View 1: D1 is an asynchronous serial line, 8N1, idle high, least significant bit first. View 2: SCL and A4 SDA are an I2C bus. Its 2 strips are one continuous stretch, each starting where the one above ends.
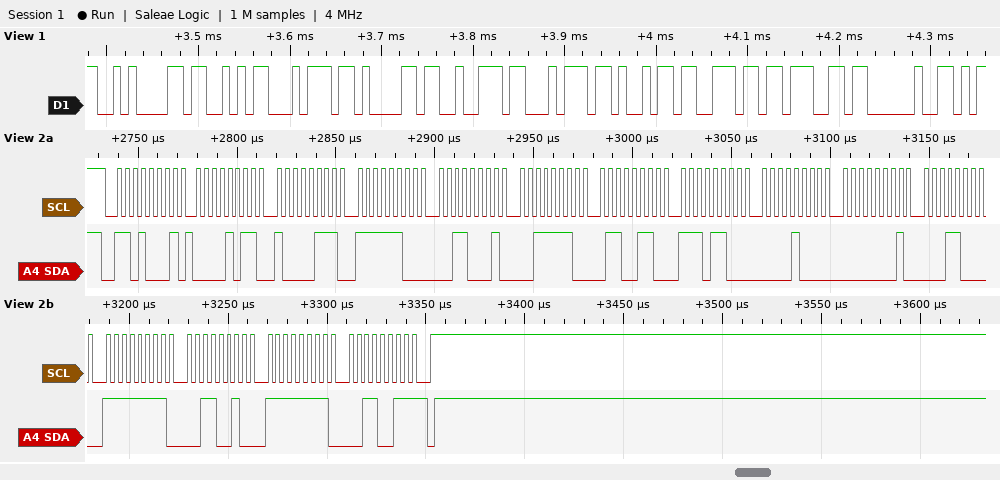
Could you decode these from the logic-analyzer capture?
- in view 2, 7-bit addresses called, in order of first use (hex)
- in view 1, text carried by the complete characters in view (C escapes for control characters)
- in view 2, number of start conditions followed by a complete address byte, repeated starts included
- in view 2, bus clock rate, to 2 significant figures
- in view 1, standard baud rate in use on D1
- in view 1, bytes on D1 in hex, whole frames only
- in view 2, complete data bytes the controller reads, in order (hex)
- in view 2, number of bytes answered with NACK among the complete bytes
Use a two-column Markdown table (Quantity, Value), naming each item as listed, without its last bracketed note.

| Quantity | Value |
|---|---|
| in view 2, 7-bit addresses called, in order of first use | 0x68 |
| in view 1, text carried by the complete characters in view | "\nStarting " |
| in view 2, number of start conditions followed by a complete address byte, repeated starts included | 1 |
| in view 2, bus clock rate, to 2 significant figures | 250 kHz |
| in view 1, standard baud rate in use on D1 | 115200 baud |
| in view 1, bytes on D1 in hex, whole frames only | 0x0A 0x53 0x74 0x61 0x72 0x74 0x69 0x6E 0x67 0x20 |
| in view 2, complete data bytes the controller reads, in order | 0B 87 FC 31 3E 66 EC 08 01 18 FF 32 FF 33 |
| in view 2, number of bytes answered with NACK among the complete bytes | 1 |
